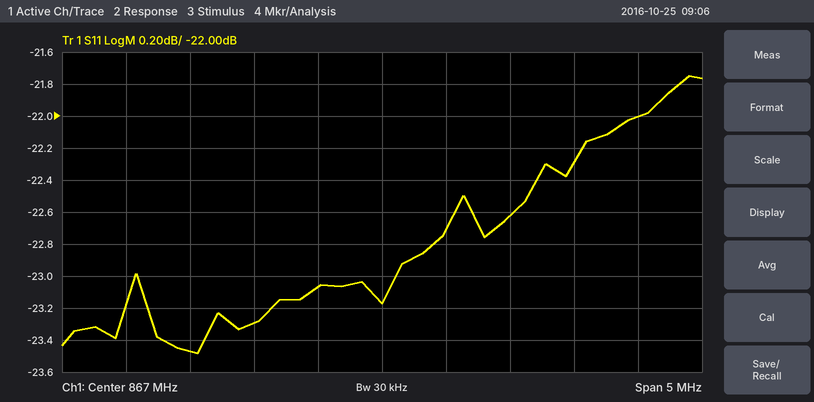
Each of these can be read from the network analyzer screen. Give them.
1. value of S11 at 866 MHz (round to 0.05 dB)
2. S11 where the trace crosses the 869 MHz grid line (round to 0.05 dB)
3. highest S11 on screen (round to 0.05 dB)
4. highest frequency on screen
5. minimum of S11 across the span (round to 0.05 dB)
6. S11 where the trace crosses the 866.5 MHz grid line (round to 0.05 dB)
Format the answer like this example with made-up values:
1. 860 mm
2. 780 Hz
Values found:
1. -23.30 dB
2. -22.00 dB
3. -21.75 dB
4. 869.5 MHz
5. -23.50 dB
6. -23.05 dB
